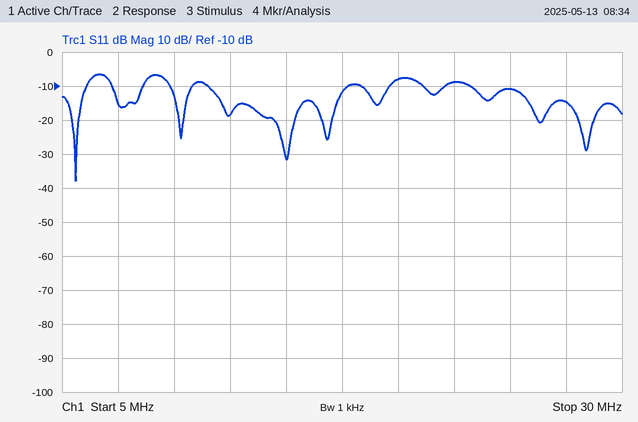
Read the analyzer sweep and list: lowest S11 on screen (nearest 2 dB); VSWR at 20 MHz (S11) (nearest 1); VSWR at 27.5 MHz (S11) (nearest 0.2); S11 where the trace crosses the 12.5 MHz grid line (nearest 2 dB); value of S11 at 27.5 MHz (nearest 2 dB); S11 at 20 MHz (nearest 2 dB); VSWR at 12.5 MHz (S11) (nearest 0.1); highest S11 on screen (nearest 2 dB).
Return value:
-38 dB
2
1.4
-18 dB
-14 dB
-8 dB
1.3
-6 dB
